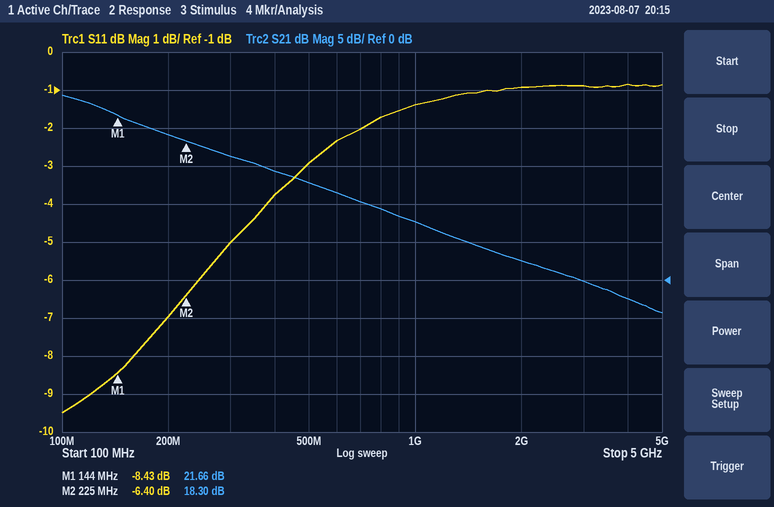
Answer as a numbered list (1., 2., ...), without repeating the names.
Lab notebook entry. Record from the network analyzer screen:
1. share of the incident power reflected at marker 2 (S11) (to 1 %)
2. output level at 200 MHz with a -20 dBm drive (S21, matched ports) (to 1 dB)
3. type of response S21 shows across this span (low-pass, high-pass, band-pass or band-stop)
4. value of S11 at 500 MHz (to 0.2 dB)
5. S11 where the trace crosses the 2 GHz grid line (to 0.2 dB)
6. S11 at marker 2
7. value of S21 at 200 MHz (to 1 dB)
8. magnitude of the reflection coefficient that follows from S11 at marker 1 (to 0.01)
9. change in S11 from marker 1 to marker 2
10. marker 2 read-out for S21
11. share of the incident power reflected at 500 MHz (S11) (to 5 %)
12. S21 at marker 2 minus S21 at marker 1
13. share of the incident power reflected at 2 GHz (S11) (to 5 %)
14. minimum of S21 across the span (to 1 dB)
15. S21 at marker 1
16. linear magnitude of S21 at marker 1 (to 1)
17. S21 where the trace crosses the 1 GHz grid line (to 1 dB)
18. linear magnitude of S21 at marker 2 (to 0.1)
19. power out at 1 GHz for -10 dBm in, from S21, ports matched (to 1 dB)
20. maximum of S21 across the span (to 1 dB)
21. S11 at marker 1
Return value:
1. 23 %
2. -1 dBm
3. low-pass
4. -3.0 dB
5. -1.0 dB
6. -6.40 dB
7. 19 dB
8. 0.38
9. 2.03 dB
10. 18.30 dB
11. 50 %
12. -3.36 dB
13. 80 %
14. -4 dB
15. 21.66 dB
16. 12
17. 8 dB
18. 8.2
19. -2 dBm
20. 24 dB
21. -8.43 dB
